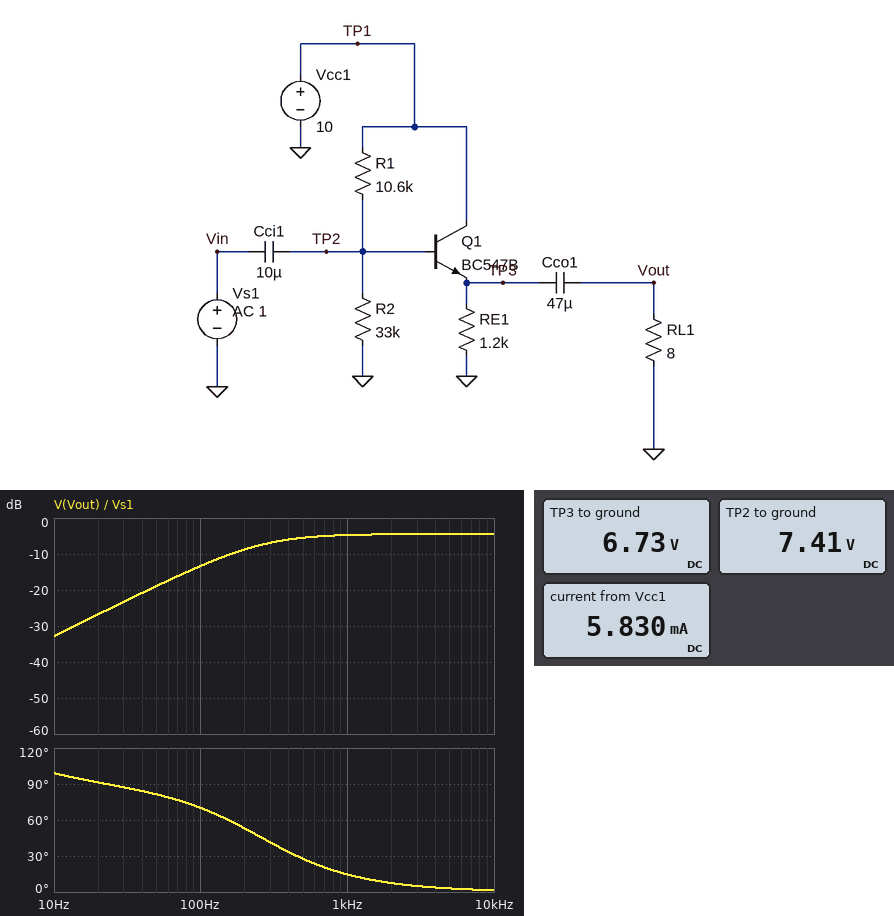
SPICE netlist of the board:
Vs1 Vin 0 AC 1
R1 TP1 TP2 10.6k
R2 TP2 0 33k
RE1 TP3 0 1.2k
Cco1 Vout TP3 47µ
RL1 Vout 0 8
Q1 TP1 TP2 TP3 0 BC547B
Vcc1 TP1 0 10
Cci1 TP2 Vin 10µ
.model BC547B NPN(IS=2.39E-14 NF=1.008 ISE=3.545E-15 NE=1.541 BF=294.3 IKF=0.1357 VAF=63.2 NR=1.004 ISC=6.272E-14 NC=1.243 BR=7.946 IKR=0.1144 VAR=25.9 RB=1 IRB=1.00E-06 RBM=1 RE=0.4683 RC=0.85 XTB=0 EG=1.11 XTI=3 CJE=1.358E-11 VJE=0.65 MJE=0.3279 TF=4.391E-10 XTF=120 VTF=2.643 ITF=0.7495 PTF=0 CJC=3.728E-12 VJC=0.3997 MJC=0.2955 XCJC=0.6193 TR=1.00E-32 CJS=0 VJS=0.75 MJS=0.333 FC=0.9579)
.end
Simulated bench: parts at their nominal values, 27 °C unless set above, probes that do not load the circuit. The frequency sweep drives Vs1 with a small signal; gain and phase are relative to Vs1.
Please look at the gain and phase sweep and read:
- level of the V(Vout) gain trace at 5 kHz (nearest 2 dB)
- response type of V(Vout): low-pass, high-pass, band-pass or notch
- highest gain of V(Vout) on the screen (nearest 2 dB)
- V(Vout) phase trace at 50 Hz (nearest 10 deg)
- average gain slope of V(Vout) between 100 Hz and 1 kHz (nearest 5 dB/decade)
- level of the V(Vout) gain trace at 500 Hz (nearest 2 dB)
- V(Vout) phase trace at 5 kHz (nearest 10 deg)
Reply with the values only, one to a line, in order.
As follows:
-4 dB
high-pass
-4 dB
80 deg
10 dB/decade
-6 dB
0 deg
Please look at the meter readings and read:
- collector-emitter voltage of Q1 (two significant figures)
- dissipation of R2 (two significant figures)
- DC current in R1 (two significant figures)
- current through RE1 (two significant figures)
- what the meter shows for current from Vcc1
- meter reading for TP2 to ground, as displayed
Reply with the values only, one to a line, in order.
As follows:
3.3 V
1.7 mW
240 µA
5.6 mA
5.830 mA
7.41 V
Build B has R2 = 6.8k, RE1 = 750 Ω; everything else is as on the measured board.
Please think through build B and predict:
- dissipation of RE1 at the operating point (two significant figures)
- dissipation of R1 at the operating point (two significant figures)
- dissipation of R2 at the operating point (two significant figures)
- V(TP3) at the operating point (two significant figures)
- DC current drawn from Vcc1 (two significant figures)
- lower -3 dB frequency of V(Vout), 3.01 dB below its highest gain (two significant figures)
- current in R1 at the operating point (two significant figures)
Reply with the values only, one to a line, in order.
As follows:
13 mW
3.6 mW
2.2 mW
3.2 V
4.8 mA
230 Hz
580 µA
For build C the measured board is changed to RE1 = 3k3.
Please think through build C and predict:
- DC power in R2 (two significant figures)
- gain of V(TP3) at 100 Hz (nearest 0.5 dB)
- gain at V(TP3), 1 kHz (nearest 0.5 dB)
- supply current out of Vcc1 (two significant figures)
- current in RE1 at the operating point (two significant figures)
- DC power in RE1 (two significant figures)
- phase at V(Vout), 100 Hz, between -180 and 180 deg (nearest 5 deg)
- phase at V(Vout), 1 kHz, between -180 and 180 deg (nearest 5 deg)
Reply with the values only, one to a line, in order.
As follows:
1.7 mW
-1.5 dB
-8.0 dB
2.3 mA
2.1 mA
14 mW
60 deg
10 deg
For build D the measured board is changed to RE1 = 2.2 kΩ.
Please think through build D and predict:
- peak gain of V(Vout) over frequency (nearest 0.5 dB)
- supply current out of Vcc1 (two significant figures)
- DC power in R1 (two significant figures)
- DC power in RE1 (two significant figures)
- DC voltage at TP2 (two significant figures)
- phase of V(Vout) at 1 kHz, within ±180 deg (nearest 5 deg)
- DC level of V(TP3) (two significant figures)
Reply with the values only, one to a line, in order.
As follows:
-6.5 dB
3.3 mA
600 µW
21 mW
7.5 V
10 deg
6.8 V
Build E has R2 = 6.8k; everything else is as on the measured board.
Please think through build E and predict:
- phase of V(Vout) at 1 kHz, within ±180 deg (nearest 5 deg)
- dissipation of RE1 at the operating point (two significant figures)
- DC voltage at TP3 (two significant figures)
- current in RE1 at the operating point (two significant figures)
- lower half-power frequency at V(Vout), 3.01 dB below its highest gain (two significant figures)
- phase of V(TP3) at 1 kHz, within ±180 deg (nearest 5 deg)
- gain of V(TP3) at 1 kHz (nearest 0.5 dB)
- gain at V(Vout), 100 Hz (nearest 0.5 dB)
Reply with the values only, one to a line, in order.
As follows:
10 deg
8.6 mW
3.2 V
2.7 mA
190 Hz
-10 deg
-6.5 dB
-14.0 dB
